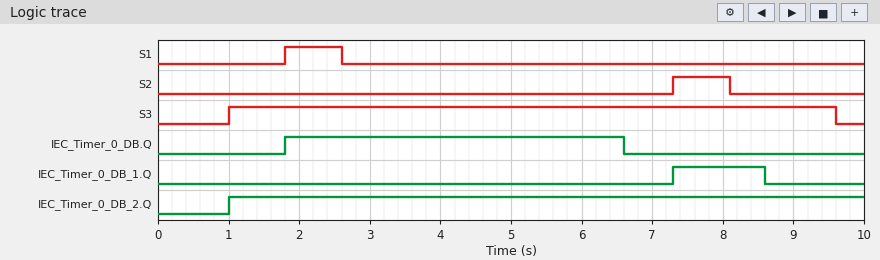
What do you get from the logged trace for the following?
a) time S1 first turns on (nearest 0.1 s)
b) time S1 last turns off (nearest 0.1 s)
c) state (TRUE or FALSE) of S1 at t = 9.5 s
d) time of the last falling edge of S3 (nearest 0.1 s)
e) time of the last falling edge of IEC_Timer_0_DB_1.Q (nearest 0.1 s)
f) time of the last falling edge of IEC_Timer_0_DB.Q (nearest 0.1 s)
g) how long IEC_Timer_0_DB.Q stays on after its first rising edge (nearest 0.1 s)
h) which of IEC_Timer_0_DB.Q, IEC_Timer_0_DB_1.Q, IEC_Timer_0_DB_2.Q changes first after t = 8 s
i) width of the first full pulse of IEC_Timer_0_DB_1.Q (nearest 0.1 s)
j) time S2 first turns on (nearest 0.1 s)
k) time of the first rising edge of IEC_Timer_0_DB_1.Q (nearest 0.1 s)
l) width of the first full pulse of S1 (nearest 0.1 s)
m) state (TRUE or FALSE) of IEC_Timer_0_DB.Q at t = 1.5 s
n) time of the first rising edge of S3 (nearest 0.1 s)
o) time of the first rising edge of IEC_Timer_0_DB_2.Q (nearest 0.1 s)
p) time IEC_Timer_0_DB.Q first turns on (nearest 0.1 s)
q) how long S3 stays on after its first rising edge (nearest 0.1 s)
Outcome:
1.8 s
2.6 s
FALSE
9.6 s
8.6 s
6.6 s
4.8 s
IEC_Timer_0_DB_1.Q
1.3 s
7.3 s
7.3 s
0.8 s
FALSE
1.0 s
1.0 s
1.8 s
8.6 s
